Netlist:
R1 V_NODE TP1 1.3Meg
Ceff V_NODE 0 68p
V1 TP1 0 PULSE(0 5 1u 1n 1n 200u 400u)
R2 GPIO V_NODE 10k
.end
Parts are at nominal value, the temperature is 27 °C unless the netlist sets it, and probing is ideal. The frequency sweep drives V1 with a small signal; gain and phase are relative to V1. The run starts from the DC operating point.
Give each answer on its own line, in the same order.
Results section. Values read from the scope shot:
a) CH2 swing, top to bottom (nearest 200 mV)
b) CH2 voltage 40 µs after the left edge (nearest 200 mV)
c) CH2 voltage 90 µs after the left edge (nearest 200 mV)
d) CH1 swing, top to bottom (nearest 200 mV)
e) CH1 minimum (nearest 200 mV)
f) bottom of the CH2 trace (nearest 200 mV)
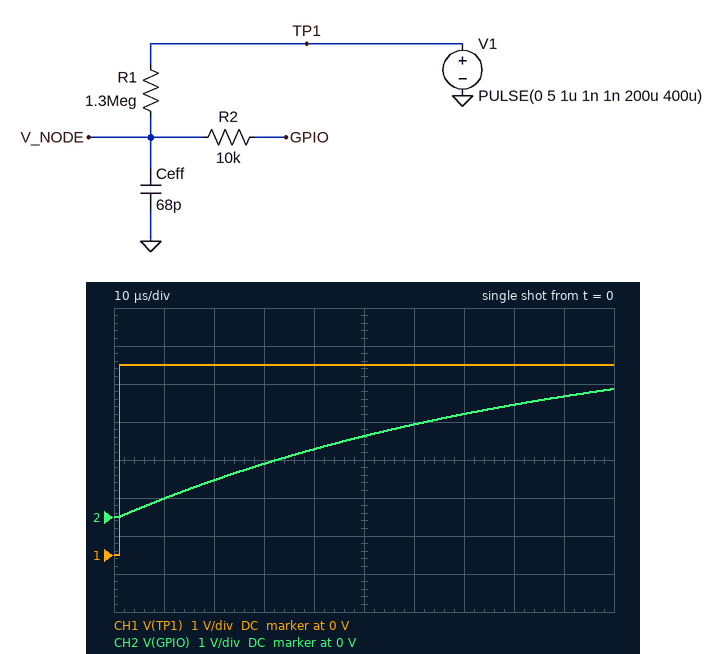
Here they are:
3.4 V
1.8 V
3.2 V
5.0 V
0 V
0 V
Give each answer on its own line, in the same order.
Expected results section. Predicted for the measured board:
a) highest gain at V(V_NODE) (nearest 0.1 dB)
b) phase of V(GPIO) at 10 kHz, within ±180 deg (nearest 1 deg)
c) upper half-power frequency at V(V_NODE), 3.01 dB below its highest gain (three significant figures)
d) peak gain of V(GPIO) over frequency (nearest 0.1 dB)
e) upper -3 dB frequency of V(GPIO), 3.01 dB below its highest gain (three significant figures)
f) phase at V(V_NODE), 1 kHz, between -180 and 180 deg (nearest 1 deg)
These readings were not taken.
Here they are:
0 dB
-80 deg
1.80 kHz
0 dB
1.80 kHz
-29 deg
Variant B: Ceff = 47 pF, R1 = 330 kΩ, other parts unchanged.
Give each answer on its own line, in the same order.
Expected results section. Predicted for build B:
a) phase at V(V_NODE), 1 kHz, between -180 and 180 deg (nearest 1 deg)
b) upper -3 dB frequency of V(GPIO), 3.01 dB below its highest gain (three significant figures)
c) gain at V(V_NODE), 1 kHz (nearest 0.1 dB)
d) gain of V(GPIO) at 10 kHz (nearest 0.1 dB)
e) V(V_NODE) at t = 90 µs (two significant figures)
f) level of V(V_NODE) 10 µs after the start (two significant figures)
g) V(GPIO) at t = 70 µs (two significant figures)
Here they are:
-6 deg
10.3 kHz
0 dB
-2.9 dB
5.0 V
2.2 V
4.9 V
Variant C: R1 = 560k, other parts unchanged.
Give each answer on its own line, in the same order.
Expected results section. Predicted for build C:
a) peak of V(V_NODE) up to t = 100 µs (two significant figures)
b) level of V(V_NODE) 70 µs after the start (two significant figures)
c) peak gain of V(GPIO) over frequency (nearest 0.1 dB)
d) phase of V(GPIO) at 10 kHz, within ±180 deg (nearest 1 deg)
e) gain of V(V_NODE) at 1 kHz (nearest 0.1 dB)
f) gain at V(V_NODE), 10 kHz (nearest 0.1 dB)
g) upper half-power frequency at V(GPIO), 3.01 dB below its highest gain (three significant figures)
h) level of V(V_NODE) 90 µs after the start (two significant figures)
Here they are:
4.6 V
4.2 V
0 dB
-67 deg
-0.2 dB
-8.3 dB
4.18 kHz
4.5 V
